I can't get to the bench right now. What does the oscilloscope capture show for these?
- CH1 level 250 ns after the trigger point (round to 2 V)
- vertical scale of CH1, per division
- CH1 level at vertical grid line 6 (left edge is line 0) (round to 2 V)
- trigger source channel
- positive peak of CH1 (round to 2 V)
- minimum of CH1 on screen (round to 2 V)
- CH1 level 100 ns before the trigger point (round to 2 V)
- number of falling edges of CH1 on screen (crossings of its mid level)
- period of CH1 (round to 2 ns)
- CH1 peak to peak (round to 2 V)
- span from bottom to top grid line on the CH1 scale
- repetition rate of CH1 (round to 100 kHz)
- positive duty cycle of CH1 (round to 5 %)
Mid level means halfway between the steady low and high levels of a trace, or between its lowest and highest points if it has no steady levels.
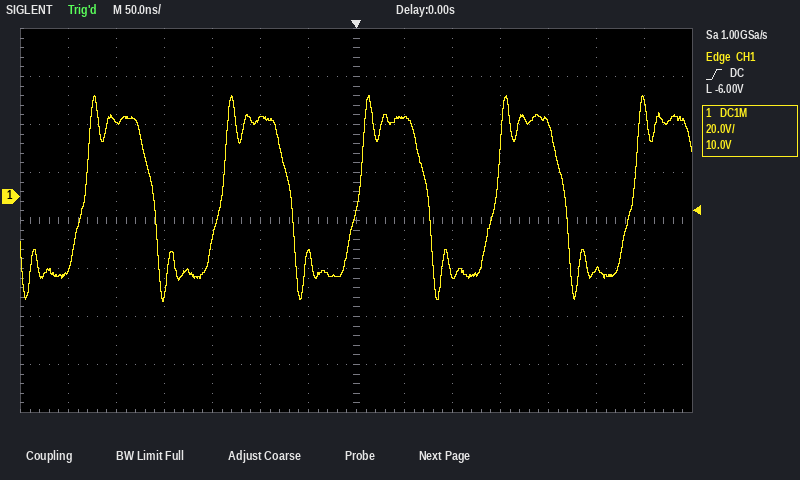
-30 V
20 V
-24 V
CH1
42 V
-44 V
32 V
4
142 ns
86 V
160 V
7.0 MHz
50 %
